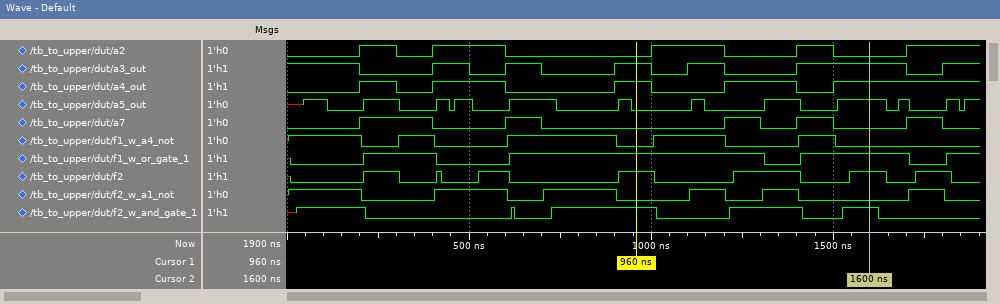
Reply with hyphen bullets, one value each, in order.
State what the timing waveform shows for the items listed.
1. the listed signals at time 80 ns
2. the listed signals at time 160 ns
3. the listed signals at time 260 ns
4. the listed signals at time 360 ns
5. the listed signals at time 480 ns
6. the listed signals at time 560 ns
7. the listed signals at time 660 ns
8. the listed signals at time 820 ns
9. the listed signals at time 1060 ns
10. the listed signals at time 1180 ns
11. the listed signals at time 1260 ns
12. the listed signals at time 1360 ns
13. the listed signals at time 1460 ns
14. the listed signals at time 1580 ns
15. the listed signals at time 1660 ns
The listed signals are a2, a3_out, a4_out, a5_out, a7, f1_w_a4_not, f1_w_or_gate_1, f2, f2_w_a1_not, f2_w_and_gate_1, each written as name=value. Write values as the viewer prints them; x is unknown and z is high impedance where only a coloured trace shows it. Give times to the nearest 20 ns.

- a2=0, a3_out=1, a4_out=0, a5_out=1, a7=0, f1_w_a4_not=1, f1_w_or_gate_1=0, f2=0, f2_w_a1_not=1, f2_w_and_gate_1=1
- a2=0, a3_out=1, a4_out=0, a5_out=0, a7=0, f1_w_a4_not=1, f1_w_or_gate_1=0, f2=0, f2_w_a1_not=1, f2_w_and_gate_1=1
- a2=1, a3_out=0, a4_out=1, a5_out=1, a7=1, f1_w_a4_not=0, f1_w_or_gate_1=1, f2=1, f2_w_a1_not=0, f2_w_and_gate_1=0
- a2=0, a3_out=0, a4_out=0, a5_out=0, a7=1, f1_w_a4_not=1, f1_w_or_gate_1=1, f2=0, f2_w_a1_not=0, f2_w_and_gate_1=0
- a2=1, a3_out=1, a4_out=1, a5_out=1, a7=0, f1_w_a4_not=0, f1_w_or_gate_1=0, f2=0, f2_w_a1_not=1, f2_w_and_gate_1=0
- a2=1, a3_out=0, a4_out=1, a5_out=0, a7=0, f1_w_a4_not=0, f1_w_or_gate_1=0, f2=1, f2_w_a1_not=1, f2_w_and_gate_1=0
- a2=0, a3_out=1, a4_out=0, a5_out=1, a7=1, f1_w_a4_not=1, f1_w_or_gate_1=1, f2=0, f2_w_a1_not=0, f2_w_and_gate_1=0
- a2=0, a3_out=0, a4_out=0, a5_out=0, a7=0, f1_w_a4_not=1, f1_w_or_gate_1=1, f2=0, f2_w_a1_not=1, f2_w_and_gate_1=1
- a2=1, a3_out=0, a4_out=0, a5_out=0, a7=0, f1_w_a4_not=1, f1_w_or_gate_1=1, f2=0, f2_w_a1_not=0, f2_w_and_gate_1=0
- a2=1, a3_out=1, a4_out=0, a5_out=0, a7=0, f1_w_a4_not=1, f1_w_or_gate_1=1, f2=0, f2_w_a1_not=1, f2_w_and_gate_1=0
- a2=0, a3_out=0, a4_out=1, a5_out=0, a7=1, f1_w_a4_not=0, f1_w_or_gate_1=1, f2=1, f2_w_a1_not=0, f2_w_and_gate_1=1
- a2=0, a3_out=0, a4_out=1, a5_out=1, a7=0, f1_w_a4_not=0, f1_w_or_gate_1=0, f2=1, f2_w_a1_not=1, f2_w_and_gate_1=1
- a2=1, a3_out=1, a4_out=0, a5_out=0, a7=1, f1_w_a4_not=1, f1_w_or_gate_1=1, f2=0, f2_w_a1_not=0, f2_w_and_gate_1=0
- a2=0, a3_out=1, a4_out=1, a5_out=1, a7=0, f1_w_a4_not=0, f1_w_or_gate_1=1, f2=1, f2_w_a1_not=0, f2_w_and_gate_1=1
- a2=0, a3_out=1, a4_out=1, a5_out=0, a7=0, f1_w_a4_not=0, f1_w_or_gate_1=1, f2=0, f2_w_a1_not=0, f2_w_and_gate_1=0
